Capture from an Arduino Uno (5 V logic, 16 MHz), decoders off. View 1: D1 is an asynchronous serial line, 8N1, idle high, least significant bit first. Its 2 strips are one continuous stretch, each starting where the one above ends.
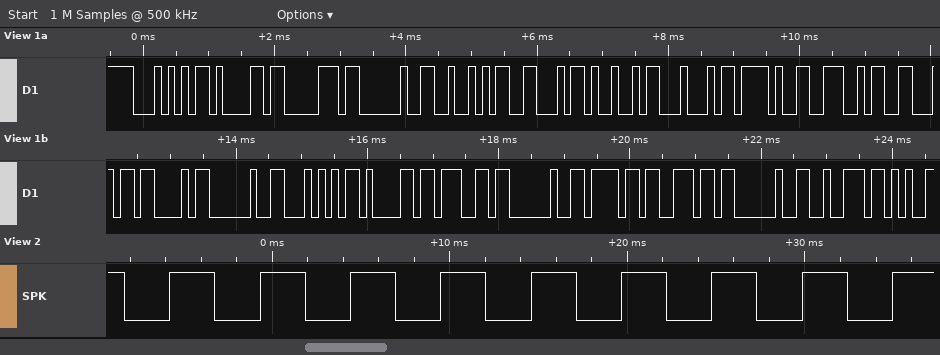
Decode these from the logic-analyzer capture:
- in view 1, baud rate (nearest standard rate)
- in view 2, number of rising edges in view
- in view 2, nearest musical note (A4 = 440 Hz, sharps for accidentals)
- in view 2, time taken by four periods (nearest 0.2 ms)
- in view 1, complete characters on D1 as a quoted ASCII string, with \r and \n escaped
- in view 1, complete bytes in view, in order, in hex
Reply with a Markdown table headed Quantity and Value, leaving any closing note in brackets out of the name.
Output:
| Quantity | Value |
|---|---|
| in view 1, baud rate | 9600 baud |
| in view 2, number of rising edges in view | 9 |
| in view 2, nearest musical note | G3 |
| in view 2, time taken by four periods | 20.4 ms |
| in view 1, complete characters on D1 as a quoted ASCII string, with \r and \n escaped | "Tap RFID/NFC Tag on r" |
| in view 1, complete bytes in view, in order, in hex | 54 61 70 20 52 46 49 44 2F 4E 46 43 20 54 61 67 20 6F 6E 20 72 |
